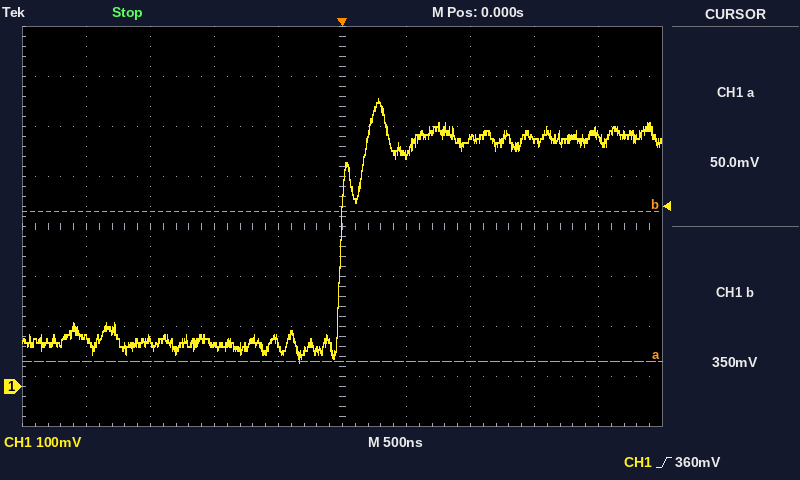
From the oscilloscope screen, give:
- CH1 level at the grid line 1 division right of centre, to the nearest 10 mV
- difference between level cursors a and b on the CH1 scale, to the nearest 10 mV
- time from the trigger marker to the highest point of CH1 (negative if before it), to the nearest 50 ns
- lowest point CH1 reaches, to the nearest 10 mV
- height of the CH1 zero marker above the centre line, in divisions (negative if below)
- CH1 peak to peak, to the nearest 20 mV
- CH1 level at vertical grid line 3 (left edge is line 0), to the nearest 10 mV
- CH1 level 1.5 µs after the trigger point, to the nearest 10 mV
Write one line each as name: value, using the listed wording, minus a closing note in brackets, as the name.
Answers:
CH1 level at the grid line 1 division right of centre, to the nearest 10 mV: 460 mV
difference between level cursors a and b on the CH1 scale, to the nearest 10 mV: 300 mV
time from the trigger marker to the highest point of CH1 (negative if before it), to the nearest 50 ns: +300 ns
lowest point CH1 reaches, to the nearest 10 mV: 50 mV
height of the CH1 zero marker above the centre line, in divisions: -3.2 div
CH1 peak to peak, to the nearest 20 mV: 520 mV
CH1 level at vertical grid line 3 (left edge is line 0), to the nearest 10 mV: 80 mV
CH1 level 1.5 µs after the trigger point, to the nearest 10 mV: 500 mV
